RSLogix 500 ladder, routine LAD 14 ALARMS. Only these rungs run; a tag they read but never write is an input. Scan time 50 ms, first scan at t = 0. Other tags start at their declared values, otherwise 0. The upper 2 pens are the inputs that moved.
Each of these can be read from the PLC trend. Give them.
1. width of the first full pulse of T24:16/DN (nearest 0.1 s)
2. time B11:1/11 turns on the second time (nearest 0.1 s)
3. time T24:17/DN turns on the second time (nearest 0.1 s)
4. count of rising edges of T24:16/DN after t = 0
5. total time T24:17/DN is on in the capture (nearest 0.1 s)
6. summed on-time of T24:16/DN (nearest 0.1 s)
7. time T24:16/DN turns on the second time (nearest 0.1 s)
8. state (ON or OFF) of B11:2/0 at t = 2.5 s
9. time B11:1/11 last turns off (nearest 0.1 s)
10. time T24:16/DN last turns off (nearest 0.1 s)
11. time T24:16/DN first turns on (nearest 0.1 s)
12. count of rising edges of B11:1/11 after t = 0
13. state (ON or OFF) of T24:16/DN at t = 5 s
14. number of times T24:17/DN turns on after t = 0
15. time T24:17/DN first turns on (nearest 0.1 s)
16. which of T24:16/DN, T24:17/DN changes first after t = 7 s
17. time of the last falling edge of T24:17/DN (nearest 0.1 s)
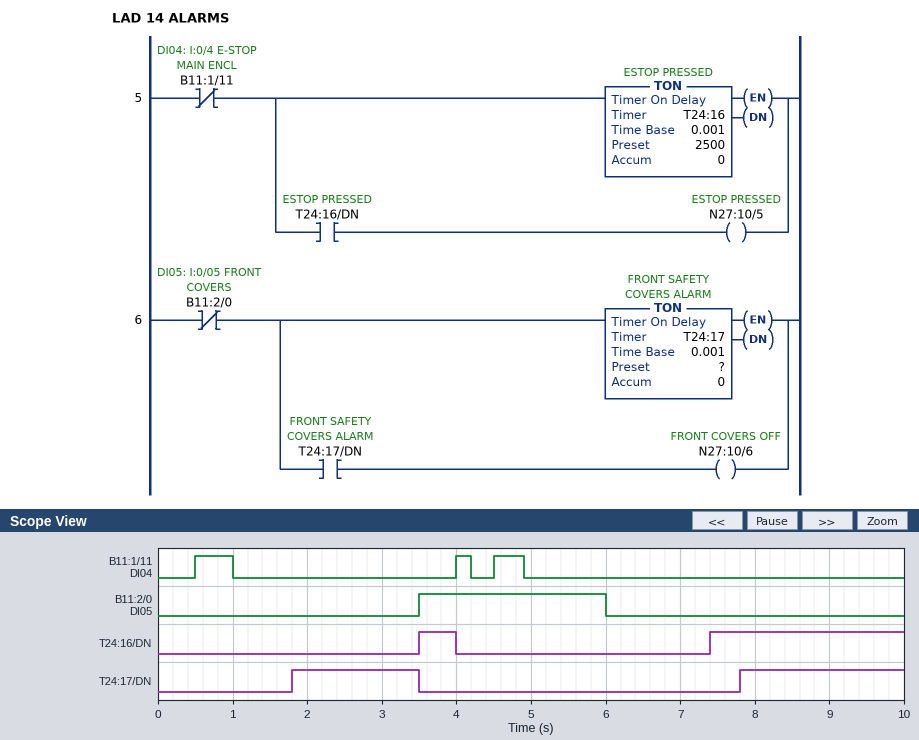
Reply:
0.5 s
4.0 s
7.8 s
2
3.9 s
3.1 s
7.4 s
OFF
4.9 s
4.0 s
3.5 s
3
OFF
2
1.8 s
T24:16/DN
3.5 s
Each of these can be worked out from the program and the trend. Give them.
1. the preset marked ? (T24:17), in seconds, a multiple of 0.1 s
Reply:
1.8 s
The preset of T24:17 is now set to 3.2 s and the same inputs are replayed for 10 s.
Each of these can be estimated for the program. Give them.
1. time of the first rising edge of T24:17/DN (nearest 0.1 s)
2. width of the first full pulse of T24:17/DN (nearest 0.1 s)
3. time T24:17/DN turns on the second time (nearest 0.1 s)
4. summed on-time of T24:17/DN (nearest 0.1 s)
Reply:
3.2 s
0.3 s
9.2 s
1.1 s
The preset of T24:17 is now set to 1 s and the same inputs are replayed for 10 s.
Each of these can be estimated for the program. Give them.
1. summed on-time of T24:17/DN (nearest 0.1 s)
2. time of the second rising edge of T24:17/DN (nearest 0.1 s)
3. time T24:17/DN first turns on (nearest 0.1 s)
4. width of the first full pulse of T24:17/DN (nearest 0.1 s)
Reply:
5.5 s
7.0 s
1.0 s
2.5 s
